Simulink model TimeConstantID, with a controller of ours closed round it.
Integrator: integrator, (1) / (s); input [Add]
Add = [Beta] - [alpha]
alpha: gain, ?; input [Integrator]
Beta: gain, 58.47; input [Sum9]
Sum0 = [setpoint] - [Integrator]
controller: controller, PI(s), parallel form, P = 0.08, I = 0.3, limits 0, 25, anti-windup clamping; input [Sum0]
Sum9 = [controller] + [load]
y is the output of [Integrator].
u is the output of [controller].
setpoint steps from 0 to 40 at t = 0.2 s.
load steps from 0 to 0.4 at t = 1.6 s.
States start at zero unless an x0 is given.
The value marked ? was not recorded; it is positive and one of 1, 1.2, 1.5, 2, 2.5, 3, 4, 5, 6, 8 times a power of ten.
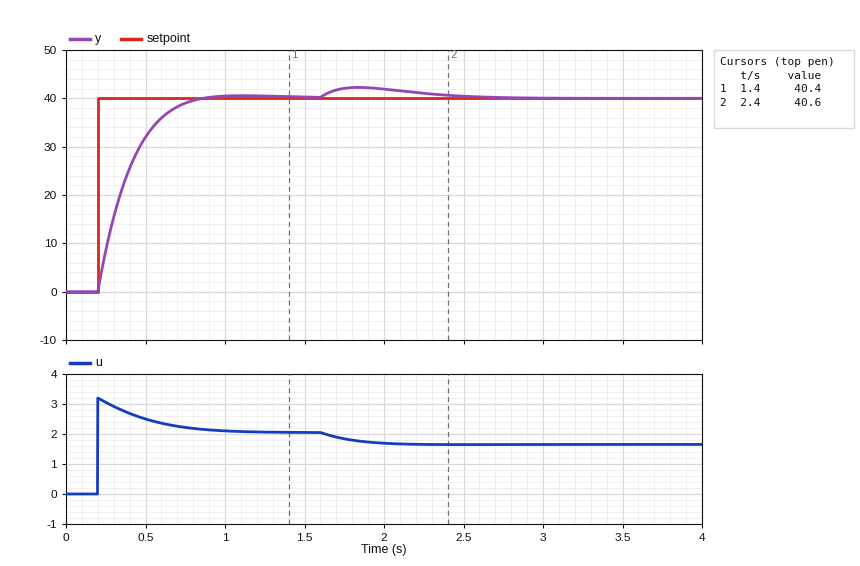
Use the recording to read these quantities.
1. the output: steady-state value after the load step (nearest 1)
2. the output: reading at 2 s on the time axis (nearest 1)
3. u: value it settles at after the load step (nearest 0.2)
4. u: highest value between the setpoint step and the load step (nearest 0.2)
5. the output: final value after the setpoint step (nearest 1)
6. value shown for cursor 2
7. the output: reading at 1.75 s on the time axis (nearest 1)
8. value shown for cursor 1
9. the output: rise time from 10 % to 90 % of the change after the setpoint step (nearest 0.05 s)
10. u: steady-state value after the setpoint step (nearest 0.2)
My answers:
40
42
1.6
3.2
40
40.6
42
40.4
0.40 s
2.0
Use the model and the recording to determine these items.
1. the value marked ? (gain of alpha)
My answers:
3
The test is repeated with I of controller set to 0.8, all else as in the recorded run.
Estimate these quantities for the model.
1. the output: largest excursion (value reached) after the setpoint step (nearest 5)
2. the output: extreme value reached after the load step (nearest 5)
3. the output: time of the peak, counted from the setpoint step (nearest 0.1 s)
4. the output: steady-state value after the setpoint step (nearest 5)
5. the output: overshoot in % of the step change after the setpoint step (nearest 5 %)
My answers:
45
40
0.4 s
40
15 %
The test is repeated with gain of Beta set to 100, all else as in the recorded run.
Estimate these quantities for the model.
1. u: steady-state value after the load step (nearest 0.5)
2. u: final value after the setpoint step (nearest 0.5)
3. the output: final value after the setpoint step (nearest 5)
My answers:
1.0
1.0
40
